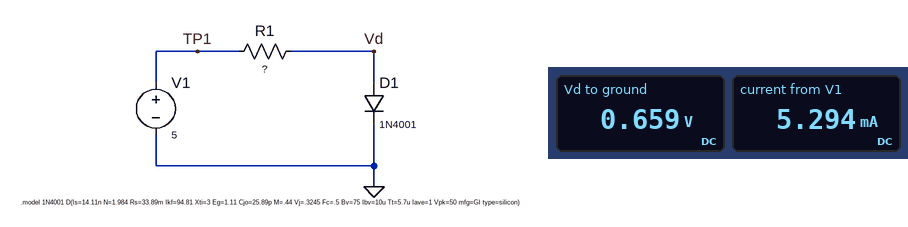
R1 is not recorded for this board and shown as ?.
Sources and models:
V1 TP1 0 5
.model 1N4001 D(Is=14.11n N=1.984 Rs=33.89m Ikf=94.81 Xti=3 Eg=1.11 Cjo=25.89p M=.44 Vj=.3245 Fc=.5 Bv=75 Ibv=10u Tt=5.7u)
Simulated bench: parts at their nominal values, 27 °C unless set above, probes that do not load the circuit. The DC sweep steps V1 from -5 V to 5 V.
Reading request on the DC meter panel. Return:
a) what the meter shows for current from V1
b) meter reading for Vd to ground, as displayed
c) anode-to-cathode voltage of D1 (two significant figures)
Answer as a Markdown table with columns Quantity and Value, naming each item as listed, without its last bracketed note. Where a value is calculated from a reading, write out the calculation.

| Quantity | Value |
|---|---|
| what the meter shows for current from V1 | 5.294 mA |
| meter reading for Vd to ground, as displayed | 0.659 V |
| anode-to-cathode voltage of D1 | 659 mV = 660 mV |
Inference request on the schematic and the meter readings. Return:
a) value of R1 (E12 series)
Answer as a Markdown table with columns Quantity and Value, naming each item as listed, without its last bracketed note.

| Quantity | Value |
|---|---|
| value of R1 | 820 Ω |
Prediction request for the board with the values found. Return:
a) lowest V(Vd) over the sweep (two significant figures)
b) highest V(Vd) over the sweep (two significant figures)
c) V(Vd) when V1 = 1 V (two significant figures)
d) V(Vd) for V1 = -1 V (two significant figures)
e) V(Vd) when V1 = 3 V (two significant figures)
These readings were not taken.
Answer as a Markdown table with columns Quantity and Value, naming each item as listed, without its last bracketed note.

| Quantity | Value |
|---|---|
| lowest V(Vd) over the sweep | -5.0 V |
| highest V(Vd) over the sweep | 660 mV |
| V(Vd) when V1 = 1 V | 540 mV |
| V(Vd) for V1 = -1 V | -1.0 V |
| V(Vd) when V1 = 3 V | 630 mV |
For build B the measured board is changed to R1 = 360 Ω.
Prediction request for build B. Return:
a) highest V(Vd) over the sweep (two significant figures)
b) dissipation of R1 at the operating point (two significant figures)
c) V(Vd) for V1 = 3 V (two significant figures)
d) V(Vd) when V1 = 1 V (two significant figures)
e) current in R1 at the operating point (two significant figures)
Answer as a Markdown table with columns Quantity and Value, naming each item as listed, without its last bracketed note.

| Quantity | Value |
|---|---|
| highest V(Vd) over the sweep | 700 mV |
| dissipation of R1 at the operating point | 51 mW |
| V(Vd) for V1 = 3 V | 670 mV |
| V(Vd) when V1 = 1 V | 580 mV |
| current in R1 at the operating point | 12 mA |
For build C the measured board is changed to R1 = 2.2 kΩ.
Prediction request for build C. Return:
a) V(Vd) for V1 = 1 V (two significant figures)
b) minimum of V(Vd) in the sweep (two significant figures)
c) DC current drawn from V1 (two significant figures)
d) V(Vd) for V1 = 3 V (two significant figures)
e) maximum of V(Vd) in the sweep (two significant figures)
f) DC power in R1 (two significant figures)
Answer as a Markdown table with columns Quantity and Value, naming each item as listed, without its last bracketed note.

| Quantity | Value |
|---|---|
| V(Vd) for V1 = 1 V | 500 mV |
| minimum of V(Vd) in the sweep | -5.0 V |
| DC current drawn from V1 | 2.0 mA |
| V(Vd) for V1 = 3 V | 580 mV |
| maximum of V(Vd) in the sweep | 610 mV |
| DC power in R1 | 8.8 mW |
